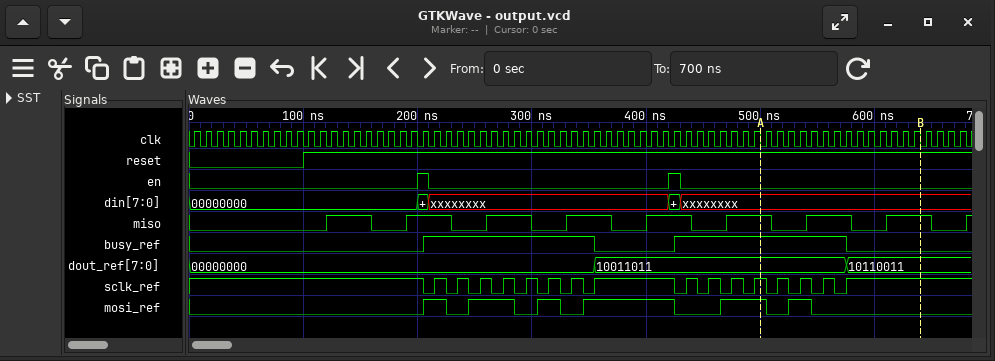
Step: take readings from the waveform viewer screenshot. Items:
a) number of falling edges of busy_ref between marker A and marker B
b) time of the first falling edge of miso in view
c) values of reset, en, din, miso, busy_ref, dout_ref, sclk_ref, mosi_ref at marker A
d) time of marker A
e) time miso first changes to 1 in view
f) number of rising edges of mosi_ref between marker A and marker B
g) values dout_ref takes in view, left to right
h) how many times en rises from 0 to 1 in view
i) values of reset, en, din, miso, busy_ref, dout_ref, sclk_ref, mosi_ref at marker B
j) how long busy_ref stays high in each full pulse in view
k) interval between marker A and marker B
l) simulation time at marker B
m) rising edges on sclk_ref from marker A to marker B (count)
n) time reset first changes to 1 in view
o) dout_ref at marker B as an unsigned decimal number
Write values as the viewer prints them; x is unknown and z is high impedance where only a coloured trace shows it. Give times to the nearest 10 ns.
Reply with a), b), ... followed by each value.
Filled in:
a) 1
b) 160 ns
c) reset=1, en=0, din=xxxxxxxx, miso=1, busy_ref=1, dout_ref=10011011, sclk_ref=1, mosi_ref=1
d) 500 ns
e) 120 ns
f) 1
g) 00000000, 10011011, 10110011
h) 2
i) reset=1, en=0, din=xxxxxxxx, miso=1, busy_ref=0, dout_ref=10110011, sclk_ref=1, mosi_ref=0
j) 150 ns, 150 ns
k) 140 ns
l) 640 ns
m) 4
n) 100 ns
o) 179
